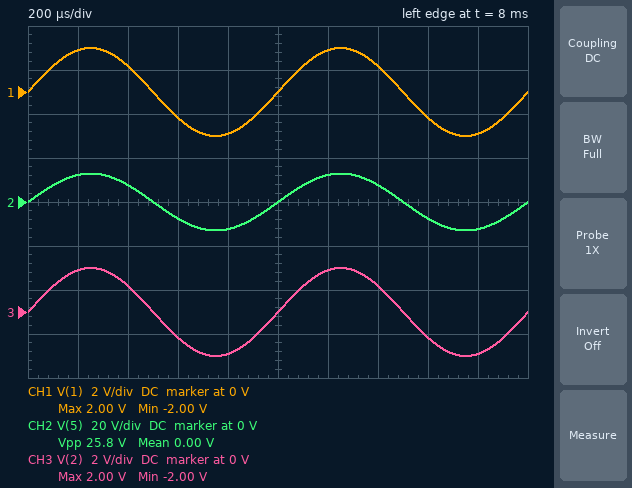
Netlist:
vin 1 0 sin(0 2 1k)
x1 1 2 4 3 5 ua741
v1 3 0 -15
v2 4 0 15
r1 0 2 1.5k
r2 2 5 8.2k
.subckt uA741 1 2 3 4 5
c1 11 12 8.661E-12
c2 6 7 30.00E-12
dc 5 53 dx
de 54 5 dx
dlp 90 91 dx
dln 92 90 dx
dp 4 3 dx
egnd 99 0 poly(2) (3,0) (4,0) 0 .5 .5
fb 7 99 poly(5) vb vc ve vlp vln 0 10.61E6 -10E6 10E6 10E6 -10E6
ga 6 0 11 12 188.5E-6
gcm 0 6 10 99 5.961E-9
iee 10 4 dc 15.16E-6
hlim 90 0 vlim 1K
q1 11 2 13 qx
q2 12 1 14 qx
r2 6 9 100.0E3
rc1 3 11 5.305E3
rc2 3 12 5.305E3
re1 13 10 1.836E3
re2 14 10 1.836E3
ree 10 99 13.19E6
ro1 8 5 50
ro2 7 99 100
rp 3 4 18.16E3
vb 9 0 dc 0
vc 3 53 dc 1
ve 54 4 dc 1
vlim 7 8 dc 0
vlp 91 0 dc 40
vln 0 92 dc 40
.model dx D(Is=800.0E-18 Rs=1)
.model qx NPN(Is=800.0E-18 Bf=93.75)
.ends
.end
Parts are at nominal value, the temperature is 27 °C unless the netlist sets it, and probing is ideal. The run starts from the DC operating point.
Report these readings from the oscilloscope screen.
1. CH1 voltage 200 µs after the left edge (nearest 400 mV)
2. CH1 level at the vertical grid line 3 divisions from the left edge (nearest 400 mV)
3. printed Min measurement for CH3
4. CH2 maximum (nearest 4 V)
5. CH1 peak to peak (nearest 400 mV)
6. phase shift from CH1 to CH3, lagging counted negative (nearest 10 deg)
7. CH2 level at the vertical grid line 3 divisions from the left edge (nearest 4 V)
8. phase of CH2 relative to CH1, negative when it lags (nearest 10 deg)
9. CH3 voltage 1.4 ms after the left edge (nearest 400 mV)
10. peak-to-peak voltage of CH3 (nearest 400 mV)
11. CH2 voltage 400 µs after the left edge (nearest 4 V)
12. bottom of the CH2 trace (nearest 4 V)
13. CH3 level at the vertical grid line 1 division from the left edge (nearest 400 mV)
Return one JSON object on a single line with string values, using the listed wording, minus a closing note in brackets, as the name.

{"CH1 voltage 200 µs after the left edge": "2.0 V", "CH1 level at the vertical grid line 3 divisions from the left edge": "-1.2 V", "printed Min measurement for CH3": "-2.00 V", "CH2 maximum": "12 V", "CH1 peak to peak": "4.0 V", "phase shift from CH1 to CH3, lagging counted negative": "0 deg", "CH2 level at the vertical grid line 3 divisions from the left edge": "-8 V", "phase of CH2 relative to CH1, negative when it lags": "0 deg", "CH3 voltage 1.4 ms after the left edge": "1.2 V", "peak-to-peak voltage of CH3": "4.0 V", "CH2 voltage 400 µs after the left edge": "8 V", "bottom of the CH2 trace": "-12 V", "CH3 level at the vertical grid line 1 division from the left edge": "2.0 V"}
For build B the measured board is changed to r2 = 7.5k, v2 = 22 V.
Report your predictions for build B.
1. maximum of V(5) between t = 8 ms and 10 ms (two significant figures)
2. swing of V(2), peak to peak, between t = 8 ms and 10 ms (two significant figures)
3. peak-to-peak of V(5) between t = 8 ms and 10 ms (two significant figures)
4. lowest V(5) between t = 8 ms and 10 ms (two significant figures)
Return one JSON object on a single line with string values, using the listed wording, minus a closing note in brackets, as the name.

{"maximum of V(5) between t = 8 ms and 10 ms": "12 V", "swing of V(2), peak to peak, between t = 8 ms and 10 ms": "4.0 V", "peak-to-peak of V(5) between t = 8 ms and 10 ms": "24 V", "lowest V(5) between t = 8 ms and 10 ms": "-12 V"}
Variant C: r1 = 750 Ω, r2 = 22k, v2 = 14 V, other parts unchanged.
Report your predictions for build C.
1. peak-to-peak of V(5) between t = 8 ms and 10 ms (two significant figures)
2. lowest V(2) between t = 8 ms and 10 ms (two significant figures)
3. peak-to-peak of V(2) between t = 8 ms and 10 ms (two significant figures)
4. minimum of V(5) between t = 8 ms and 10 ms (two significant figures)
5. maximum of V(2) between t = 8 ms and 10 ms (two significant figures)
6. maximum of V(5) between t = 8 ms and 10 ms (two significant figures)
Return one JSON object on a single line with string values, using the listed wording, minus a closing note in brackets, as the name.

{"peak-to-peak of V(5) between t = 8 ms and 10 ms": "28 V", "lowest V(2) between t = 8 ms and 10 ms": "-480 mV", "peak-to-peak of V(2) between t = 8 ms and 10 ms": "930 mV", "minimum of V(5) between t = 8 ms and 10 ms": "-15 V", "maximum of V(2) between t = 8 ms and 10 ms": "450 mV", "maximum of V(5) between t = 8 ms and 10 ms": "14 V"}
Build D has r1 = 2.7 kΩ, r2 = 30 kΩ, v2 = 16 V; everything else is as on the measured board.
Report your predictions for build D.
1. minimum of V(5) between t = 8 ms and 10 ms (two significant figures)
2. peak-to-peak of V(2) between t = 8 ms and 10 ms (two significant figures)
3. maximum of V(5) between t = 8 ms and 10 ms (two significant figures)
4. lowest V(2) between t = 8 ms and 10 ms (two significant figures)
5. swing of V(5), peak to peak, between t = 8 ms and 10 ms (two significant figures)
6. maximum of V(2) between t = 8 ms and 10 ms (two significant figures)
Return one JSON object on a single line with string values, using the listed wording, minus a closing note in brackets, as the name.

{"minimum of V(5) between t = 8 ms and 10 ms": "-15 V", "peak-to-peak of V(2) between t = 8 ms and 10 ms": "2.5 V", "maximum of V(5) between t = 8 ms and 10 ms": "16 V", "lowest V(2) between t = 8 ms and 10 ms": "-1.2 V", "swing of V(5), peak to peak, between t = 8 ms and 10 ms": "30 V", "maximum of V(2) between t = 8 ms and 10 ms": "1.3 V"}
